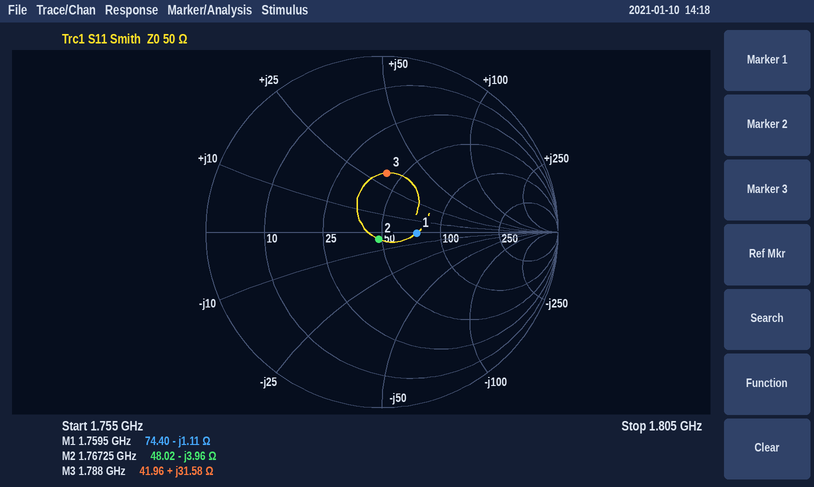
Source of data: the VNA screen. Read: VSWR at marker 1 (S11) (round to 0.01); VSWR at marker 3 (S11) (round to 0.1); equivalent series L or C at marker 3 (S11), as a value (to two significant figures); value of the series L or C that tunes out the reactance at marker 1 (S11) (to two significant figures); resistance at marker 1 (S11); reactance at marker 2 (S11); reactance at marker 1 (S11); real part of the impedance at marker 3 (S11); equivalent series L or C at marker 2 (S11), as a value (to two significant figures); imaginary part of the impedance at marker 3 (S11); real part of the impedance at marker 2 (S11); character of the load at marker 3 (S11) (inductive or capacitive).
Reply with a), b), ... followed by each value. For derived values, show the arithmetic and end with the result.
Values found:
a) 1.49
b) 2.0
c) L = 31.58 Ω/(2π × 1.788 GHz) ≈ 2.8 nH
d) L = 1.11 Ω/(2π × 1.7595 GHz) ≈ 100 pH
e) 74.40 Ω
f) -3.96 Ω
g) -1.11 Ω
h) 41.96 Ω
i) C = 1/(2π × 1.76725 GHz × 3.96 Ω) ≈ 23 pF
j) +31.58 Ω
k) 48.02 Ω
l) inductive
